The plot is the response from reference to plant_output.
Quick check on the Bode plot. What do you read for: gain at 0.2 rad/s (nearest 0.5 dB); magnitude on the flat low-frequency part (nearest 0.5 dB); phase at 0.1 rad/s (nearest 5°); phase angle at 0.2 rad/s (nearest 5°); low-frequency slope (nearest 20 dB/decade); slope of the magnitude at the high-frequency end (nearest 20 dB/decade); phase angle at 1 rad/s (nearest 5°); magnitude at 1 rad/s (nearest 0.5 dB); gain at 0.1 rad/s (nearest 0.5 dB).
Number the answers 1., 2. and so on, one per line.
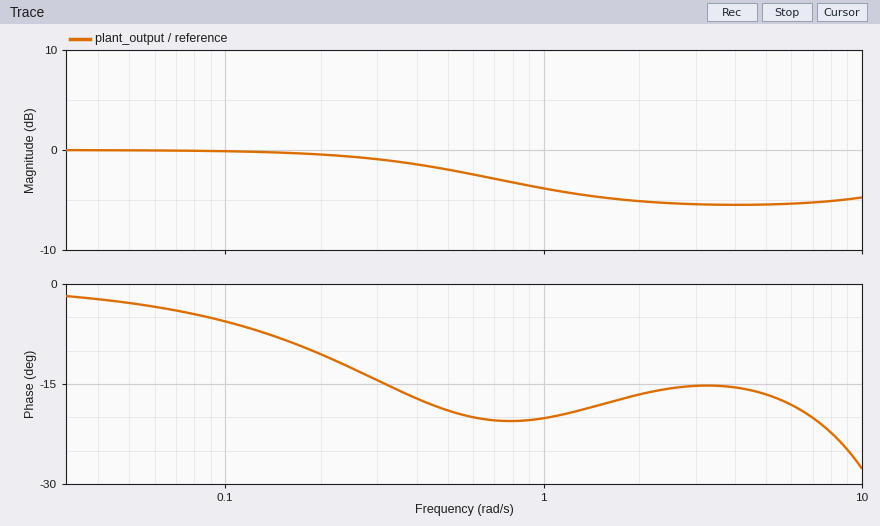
1. -0.5 dB
2. 0.0 dB
3. -5°
4. -10°
5. 0 dB/decade
6. 0 dB/decade
7. -20°
8. -4.0 dB
9. 0.0 dB
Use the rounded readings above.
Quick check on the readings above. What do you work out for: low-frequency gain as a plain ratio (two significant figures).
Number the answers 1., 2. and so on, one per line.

1. 1.0
